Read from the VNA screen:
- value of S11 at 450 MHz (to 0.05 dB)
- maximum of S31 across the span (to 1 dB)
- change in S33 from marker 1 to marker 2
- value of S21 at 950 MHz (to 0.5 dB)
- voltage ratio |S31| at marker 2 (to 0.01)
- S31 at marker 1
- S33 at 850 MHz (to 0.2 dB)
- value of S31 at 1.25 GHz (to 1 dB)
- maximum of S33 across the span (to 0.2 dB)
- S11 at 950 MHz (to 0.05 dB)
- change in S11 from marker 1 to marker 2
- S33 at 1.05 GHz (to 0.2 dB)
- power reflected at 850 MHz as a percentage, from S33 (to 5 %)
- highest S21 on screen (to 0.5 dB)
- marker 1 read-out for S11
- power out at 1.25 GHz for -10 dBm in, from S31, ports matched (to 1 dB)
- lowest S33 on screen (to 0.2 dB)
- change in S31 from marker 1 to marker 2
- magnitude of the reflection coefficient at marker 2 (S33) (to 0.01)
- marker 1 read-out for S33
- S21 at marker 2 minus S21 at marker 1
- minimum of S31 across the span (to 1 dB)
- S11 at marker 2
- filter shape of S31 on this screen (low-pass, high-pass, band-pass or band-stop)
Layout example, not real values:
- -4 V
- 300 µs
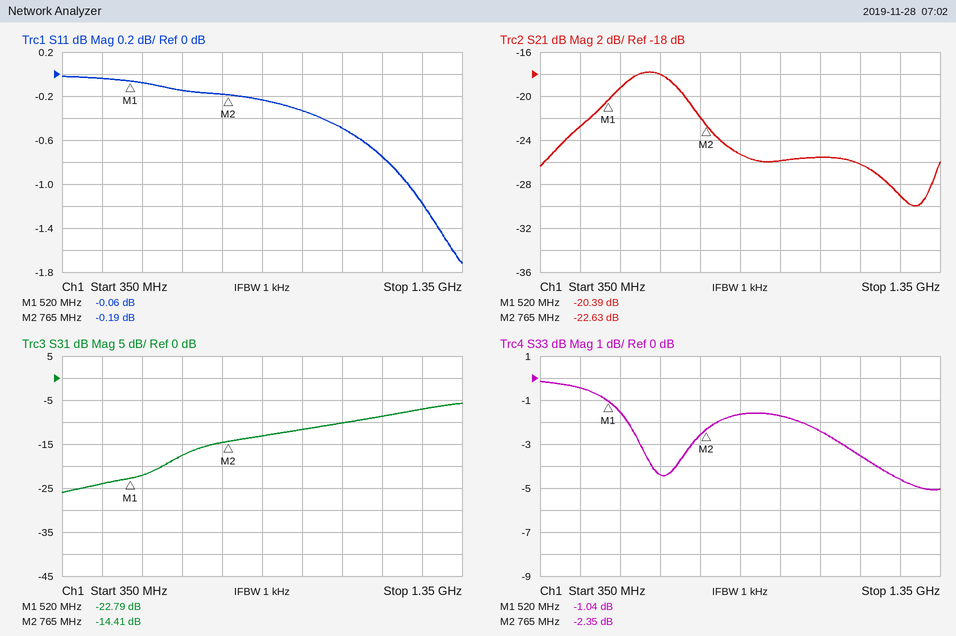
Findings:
- -0.05 dB
- -6 dB
- -1.31 dB
- -26.0 dB
- 0.19
- -22.79 dB
- -1.6 dB
- -7 dB
- -0.2 dB
- -0.35 dB
- -0.13 dB
- -2.4 dB
- 70 %
- -18.0 dB
- -0.06 dB
- -17 dBm
- -5.0 dB
- 8.38 dB
- 0.76
- -1.04 dB
- -2.24 dB
- -26 dB
- -0.19 dB
- high-pass
